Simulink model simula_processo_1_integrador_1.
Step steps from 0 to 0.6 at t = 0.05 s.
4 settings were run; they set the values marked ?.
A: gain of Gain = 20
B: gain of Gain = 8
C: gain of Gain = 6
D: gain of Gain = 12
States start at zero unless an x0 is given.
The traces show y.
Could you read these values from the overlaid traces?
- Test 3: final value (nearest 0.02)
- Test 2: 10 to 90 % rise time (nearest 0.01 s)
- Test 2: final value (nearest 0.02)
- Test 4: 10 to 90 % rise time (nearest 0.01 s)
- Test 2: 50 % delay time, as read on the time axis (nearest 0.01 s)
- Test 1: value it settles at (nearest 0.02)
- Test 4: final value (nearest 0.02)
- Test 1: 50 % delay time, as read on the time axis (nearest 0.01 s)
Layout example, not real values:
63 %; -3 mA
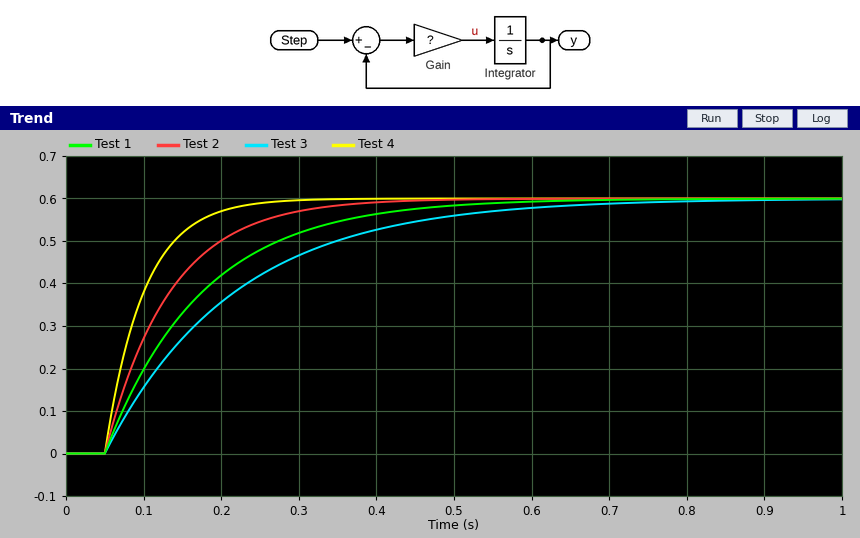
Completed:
0.60; 0.18 s; 0.60; 0.11 s; 0.11 s; 0.60; 0.60; 0.14 s
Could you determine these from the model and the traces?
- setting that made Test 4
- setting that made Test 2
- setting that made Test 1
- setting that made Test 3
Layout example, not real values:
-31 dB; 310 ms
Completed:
A; D; B; C
